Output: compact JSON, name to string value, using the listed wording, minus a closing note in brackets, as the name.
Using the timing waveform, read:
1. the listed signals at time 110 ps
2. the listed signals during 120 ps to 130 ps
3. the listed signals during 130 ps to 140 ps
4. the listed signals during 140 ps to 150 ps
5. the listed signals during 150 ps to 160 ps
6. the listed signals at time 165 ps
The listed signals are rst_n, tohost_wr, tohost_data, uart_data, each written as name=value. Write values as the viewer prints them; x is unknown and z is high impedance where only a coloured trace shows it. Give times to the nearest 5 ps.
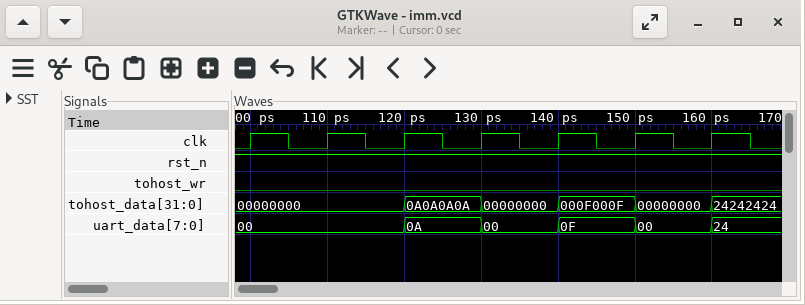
{"the listed signals at time 110 ps": "rst_n=1, tohost_wr=0, tohost_data=00000000, uart_data=00", "the listed signals during 120 ps to 130 ps": "rst_n=1, tohost_wr=0, tohost_data=0A0A0A0A, uart_data=0A", "the listed signals during 130 ps to 140 ps": "rst_n=1, tohost_wr=0, tohost_data=00000000, uart_data=00", "the listed signals during 140 ps to 150 ps": "rst_n=1, tohost_wr=0, tohost_data=000F000F, uart_data=0F", "the listed signals during 150 ps to 160 ps": "rst_n=1, tohost_wr=0, tohost_data=00000000, uart_data=00", "the listed signals at time 165 ps": "rst_n=1, tohost_wr=0, tohost_data=24242424, uart_data=24"}
